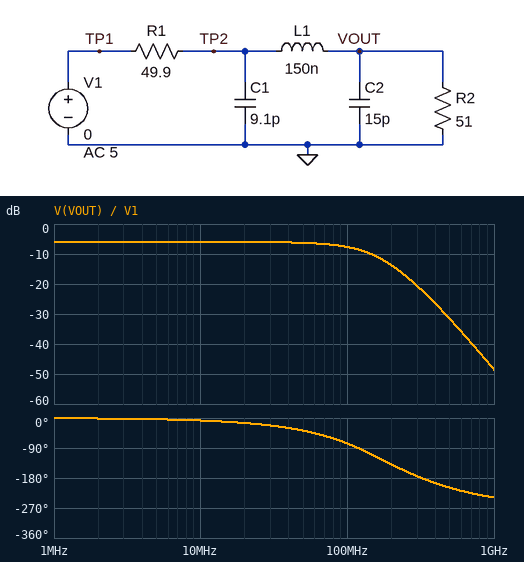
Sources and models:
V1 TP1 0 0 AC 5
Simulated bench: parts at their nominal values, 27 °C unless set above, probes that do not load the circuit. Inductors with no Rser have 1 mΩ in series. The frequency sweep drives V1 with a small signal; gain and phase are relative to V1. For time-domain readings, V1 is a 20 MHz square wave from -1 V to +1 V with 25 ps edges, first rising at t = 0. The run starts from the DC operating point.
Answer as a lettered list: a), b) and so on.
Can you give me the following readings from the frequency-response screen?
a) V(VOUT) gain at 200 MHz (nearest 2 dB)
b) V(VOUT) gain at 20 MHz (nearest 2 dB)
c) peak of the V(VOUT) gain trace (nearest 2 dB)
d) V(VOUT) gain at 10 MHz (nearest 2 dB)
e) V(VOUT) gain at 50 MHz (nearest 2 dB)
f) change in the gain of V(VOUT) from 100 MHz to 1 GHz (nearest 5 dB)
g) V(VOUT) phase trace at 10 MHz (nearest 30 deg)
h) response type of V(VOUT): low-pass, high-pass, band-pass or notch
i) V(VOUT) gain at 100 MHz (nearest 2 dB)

a) -14 dB
b) -6 dB
c) -6 dB
d) -6 dB
e) -6 dB
f) -40 dB
g) 0 deg
h) low-pass
i) -8 dB
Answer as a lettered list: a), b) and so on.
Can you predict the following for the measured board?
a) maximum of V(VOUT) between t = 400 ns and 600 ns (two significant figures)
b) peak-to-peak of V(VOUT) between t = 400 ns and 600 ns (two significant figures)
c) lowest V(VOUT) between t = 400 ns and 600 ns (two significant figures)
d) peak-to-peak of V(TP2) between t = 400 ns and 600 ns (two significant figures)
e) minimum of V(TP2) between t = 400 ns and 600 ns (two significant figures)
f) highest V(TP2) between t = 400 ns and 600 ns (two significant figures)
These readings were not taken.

a) 520 mV
b) 1.0 V
c) -520 mV
d) 2.2 V
e) -1.1 V
f) 1.1 V
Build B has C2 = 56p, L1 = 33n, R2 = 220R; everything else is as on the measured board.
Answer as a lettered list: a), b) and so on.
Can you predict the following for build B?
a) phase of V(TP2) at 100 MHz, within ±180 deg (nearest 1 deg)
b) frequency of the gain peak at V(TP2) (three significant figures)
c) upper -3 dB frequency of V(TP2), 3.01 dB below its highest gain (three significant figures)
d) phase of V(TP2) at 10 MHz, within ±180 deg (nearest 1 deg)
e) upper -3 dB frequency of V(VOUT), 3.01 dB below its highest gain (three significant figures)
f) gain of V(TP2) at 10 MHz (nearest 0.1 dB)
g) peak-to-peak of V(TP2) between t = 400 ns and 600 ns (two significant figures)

a) -57 deg
b) 315 MHz
c) 524 MHz
d) -9 deg
e) 77.1 MHz
f) -1.9 dB
g) 1.6 V
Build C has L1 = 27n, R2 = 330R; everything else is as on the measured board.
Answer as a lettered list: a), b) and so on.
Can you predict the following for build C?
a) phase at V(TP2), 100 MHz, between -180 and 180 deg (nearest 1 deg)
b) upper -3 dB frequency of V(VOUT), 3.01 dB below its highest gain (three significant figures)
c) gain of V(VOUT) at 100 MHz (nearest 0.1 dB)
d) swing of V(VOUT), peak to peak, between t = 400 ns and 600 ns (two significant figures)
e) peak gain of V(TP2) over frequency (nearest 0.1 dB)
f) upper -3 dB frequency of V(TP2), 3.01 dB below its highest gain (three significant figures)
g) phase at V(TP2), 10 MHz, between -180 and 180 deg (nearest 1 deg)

a) -34 deg
b) 396 MHz
c) -1.9 dB
d) 1.9 V
e) -0.4 dB
f) 594 MHz
g) -4 deg
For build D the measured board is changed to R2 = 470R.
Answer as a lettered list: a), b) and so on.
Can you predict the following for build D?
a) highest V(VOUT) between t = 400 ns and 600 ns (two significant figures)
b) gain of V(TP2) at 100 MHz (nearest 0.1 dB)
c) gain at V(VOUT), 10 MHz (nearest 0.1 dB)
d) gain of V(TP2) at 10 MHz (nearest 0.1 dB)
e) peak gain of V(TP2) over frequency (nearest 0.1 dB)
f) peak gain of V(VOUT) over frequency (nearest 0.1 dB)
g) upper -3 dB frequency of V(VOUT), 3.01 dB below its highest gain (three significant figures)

a) 1.5 V
b) -9.9 dB
c) -0.8 dB
d) -0.9 dB
e) -0.3 dB
f) 2.9 dB
g) 141 MHz
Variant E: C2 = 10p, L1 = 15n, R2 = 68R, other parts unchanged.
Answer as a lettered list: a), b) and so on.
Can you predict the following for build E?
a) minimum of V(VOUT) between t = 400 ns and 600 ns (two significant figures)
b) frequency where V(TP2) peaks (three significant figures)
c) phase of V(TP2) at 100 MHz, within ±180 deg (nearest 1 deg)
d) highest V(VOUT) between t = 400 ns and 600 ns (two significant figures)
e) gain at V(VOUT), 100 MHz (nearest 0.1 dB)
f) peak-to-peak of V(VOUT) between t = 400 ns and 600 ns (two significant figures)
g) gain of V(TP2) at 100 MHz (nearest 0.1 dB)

a) -660 mV
b) 629 MHz
c) -15 deg
d) 660 mV
e) -5.0 dB
f) 1.3 V
g) -5.5 dB
